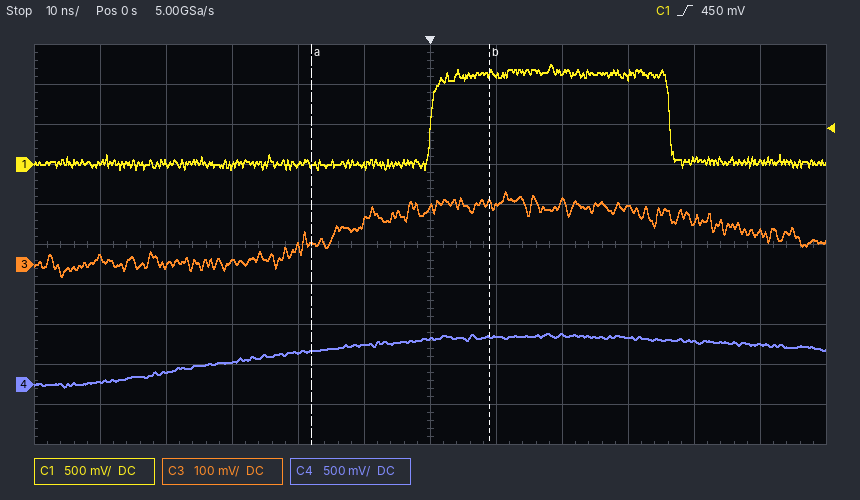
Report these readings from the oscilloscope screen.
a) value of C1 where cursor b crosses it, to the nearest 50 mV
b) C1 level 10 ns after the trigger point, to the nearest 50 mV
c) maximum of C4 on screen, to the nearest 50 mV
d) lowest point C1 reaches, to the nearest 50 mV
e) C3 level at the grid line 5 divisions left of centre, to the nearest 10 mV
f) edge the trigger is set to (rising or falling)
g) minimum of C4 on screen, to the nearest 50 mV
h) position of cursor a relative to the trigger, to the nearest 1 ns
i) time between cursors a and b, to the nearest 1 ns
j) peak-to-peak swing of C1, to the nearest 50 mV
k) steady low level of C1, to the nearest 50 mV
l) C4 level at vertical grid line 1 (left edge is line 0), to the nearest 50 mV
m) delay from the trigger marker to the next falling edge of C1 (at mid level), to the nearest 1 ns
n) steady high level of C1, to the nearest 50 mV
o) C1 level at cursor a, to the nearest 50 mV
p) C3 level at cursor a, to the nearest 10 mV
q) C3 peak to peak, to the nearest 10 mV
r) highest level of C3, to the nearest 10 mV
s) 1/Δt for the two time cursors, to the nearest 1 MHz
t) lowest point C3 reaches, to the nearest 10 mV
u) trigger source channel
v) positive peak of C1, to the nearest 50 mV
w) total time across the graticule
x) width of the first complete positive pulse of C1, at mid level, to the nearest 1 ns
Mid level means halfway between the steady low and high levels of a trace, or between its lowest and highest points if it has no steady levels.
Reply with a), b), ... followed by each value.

a) 1.15 V
b) 1.10 V
c) 650 mV
d) -50 mV
e) 20 mV
f) rising
g) -50 mV
h) -18 ns
i) 27 ns
j) 1.30 V
k) 0 mV
l) 50 mV
m) 36 ns
n) 1.15 V
o) 0 mV
p) 50 mV
q) 210 mV
r) 180 mV
s) 37 MHz
t) -30 mV
u) C1
v) 1.25 V
w) 120 ns
x) 36 ns
